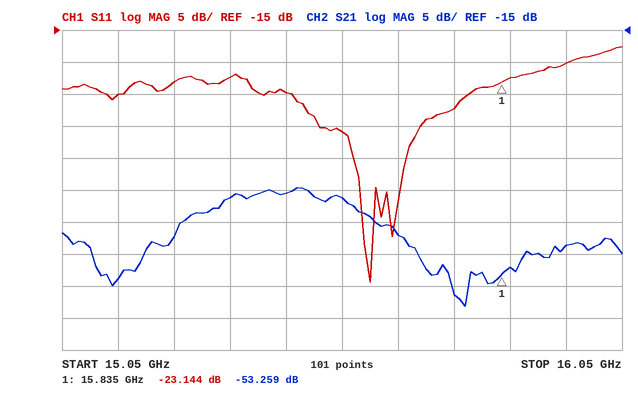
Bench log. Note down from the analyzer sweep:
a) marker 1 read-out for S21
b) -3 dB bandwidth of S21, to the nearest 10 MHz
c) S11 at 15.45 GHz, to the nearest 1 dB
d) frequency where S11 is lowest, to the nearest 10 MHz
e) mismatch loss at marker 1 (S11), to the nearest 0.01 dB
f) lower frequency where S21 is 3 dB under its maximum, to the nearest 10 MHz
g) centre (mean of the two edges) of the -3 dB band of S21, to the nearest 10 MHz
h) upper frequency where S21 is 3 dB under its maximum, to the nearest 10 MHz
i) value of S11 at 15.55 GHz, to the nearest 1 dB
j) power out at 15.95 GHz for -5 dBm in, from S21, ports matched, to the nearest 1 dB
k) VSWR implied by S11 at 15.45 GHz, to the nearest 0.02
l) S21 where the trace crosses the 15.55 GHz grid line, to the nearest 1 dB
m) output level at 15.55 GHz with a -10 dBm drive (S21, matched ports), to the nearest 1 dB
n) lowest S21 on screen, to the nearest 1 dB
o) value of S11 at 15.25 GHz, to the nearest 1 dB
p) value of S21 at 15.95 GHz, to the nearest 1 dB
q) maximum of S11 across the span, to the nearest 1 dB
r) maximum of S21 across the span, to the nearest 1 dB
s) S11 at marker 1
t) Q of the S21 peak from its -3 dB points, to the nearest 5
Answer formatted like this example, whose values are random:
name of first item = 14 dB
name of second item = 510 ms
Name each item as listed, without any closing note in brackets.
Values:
marker 1 read-out for S21 = -53.259 dB
-3 dB bandwidth of S21, to the nearest 10 MHz = 240 MHz
S11 at 15.45 GHz, to the nearest 1 dB = -25 dB
frequency where S11 is lowest, to the nearest 10 MHz = 15.60 GHz
mismatch loss at marker 1 (S11), to the nearest 0.01 dB = 0.02 dB
lower frequency where S21 is 3 dB under its maximum, to the nearest 10 MHz = 15.33 GHz
centre (mean of the two edges) of the -3 dB band of S21, to the nearest 10 MHz = 15.45 GHz
upper frequency where S21 is 3 dB under its maximum, to the nearest 10 MHz = 15.57 GHz
value of S11 at 15.55 GHz, to the nearest 1 dB = -31 dB
power out at 15.95 GHz for -5 dBm in, from S21, ports matched, to the nearest 1 dB = -54 dBm
VSWR implied by S11 at 15.45 GHz, to the nearest 0.02 = 1.12
S21 where the trace crosses the 15.55 GHz grid line, to the nearest 1 dB = -41 dB
output level at 15.55 GHz with a -10 dBm drive (S21, matched ports), to the nearest 1 dB = -51 dBm
lowest S21 on screen, to the nearest 1 dB = -58 dB
value of S11 at 15.25 GHz, to the nearest 1 dB = -23 dB
value of S21 at 15.95 GHz, to the nearest 1 dB = -49 dB
maximum of S11 across the span, to the nearest 1 dB = -18 dB
maximum of S21 across the span, to the nearest 1 dB = -40 dB
S11 at marker 1 = -23.144 dB
Q of the S21 peak from its -3 dB points, to the nearest 5 = 65
